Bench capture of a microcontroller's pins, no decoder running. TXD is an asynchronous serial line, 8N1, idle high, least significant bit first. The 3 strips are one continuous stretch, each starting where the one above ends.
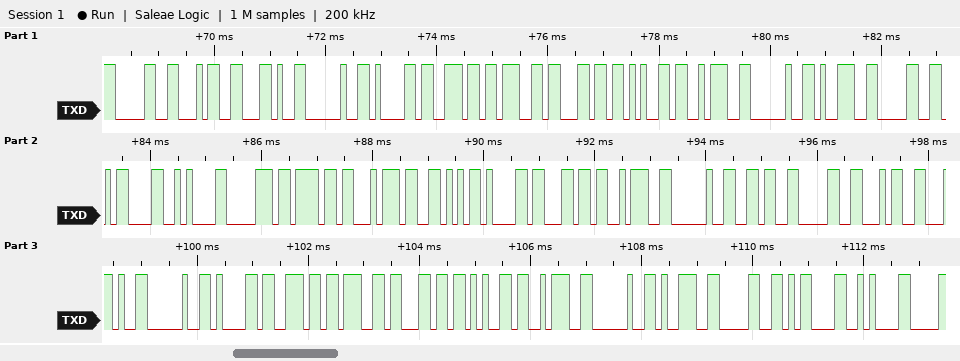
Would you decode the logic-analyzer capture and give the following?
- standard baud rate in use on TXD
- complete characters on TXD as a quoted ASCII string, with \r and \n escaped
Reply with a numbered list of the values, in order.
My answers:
1. 9600 baud
2. "04, angle: 90\r\npotVal: 604, angle: 90\r\n"
